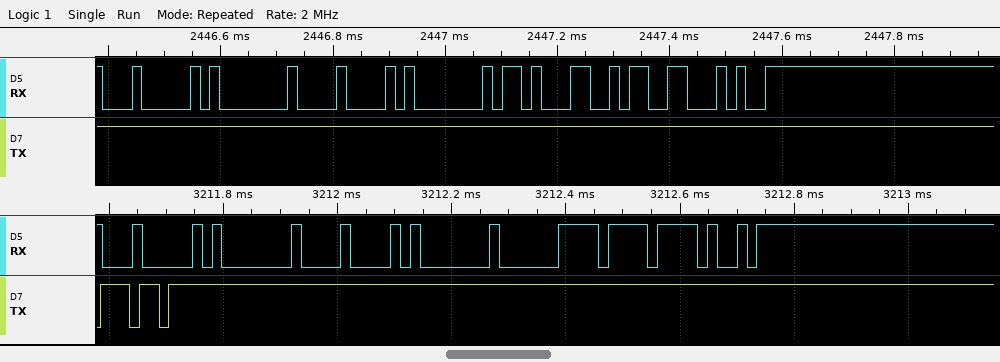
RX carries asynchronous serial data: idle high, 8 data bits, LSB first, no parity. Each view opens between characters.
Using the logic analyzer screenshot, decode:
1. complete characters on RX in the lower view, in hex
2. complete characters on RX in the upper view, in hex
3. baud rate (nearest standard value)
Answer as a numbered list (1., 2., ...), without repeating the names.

1. 04, 01, 08, 01, E0, EF, E9
2. 04, 01, 08, 01, 8B, 9A, 94
3. 57600 baud
